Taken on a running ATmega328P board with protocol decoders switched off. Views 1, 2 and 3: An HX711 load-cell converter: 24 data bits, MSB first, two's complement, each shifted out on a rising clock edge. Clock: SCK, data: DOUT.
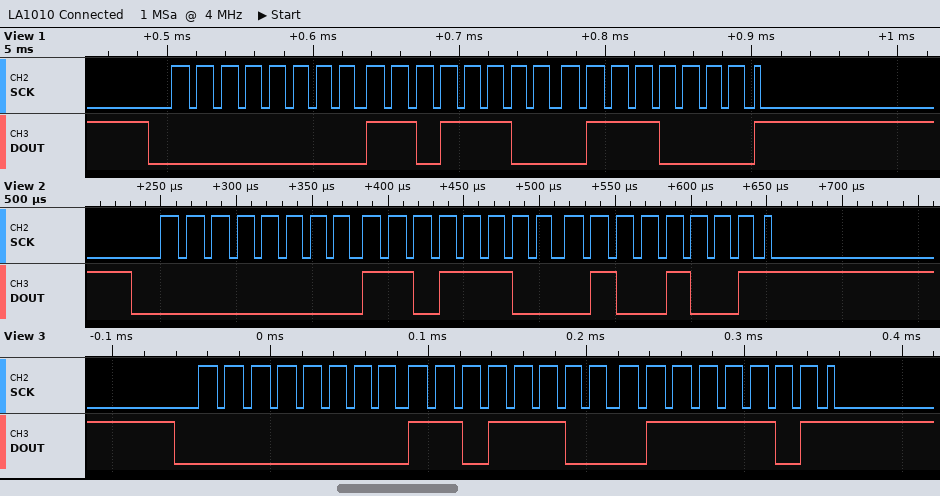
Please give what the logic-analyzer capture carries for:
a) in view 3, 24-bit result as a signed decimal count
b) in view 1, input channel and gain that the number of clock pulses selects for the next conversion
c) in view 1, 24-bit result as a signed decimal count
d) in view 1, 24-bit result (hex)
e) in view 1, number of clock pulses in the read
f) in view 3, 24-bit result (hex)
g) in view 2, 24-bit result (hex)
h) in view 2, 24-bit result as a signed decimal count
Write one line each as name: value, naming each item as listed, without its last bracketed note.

in view 3, 24-bit result as a signed decimal count: 56445
in view 1, input channel and gain that the number of clock pulses selects for the next conversion: channel A, gain 128
in view 1, 24-bit result as a signed decimal count: 56432
in view 1, 24-bit result: 0x00DC70
in view 1, number of clock pulses in the read: 25
in view 3, 24-bit result: 0x00DC7D
in view 2, 24-bit result: 0x00DC49
in view 2, 24-bit result as a signed decimal count: 56393
